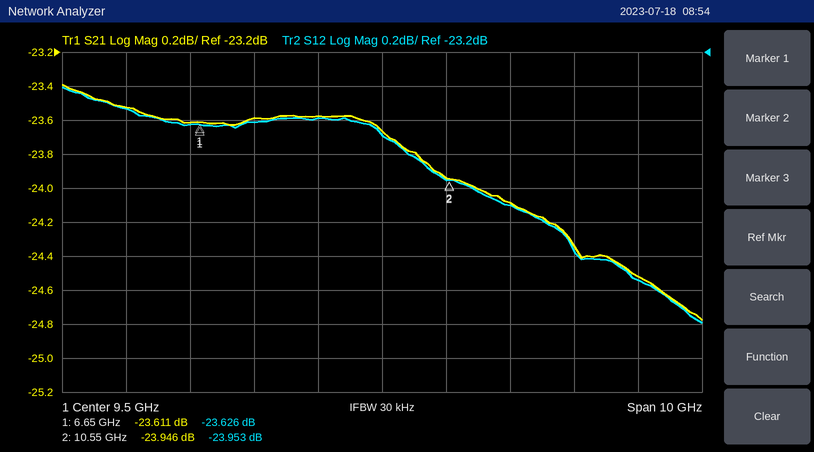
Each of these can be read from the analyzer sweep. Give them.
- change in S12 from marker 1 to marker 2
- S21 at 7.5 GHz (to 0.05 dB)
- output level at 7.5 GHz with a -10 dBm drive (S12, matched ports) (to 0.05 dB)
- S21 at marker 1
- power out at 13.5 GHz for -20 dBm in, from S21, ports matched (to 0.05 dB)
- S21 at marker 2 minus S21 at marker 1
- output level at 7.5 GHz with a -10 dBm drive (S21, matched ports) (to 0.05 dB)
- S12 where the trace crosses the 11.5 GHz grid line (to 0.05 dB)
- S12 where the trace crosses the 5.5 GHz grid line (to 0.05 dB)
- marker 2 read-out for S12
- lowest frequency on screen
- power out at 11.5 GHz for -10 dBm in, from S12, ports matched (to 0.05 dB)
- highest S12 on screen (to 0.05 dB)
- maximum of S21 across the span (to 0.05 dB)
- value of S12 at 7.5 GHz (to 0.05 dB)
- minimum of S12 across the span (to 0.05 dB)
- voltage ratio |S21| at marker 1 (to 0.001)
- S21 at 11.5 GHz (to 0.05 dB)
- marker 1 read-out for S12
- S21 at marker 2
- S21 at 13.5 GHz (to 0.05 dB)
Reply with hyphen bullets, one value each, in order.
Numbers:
- -0.327 dB
- -23.60 dB
- -33.60 dBm
- -23.611 dB
- -44.50 dBm
- -0.335 dB
- -33.60 dBm
- -24.10 dB
- -23.55 dB
- -23.953 dB
- 4.5 GHz
- -34.10 dBm
- -23.40 dB
- -23.40 dB
- -23.60 dB
- -24.80 dB
- 0.066
- -24.10 dB
- -23.626 dB
- -23.946 dB
- -24.50 dB
